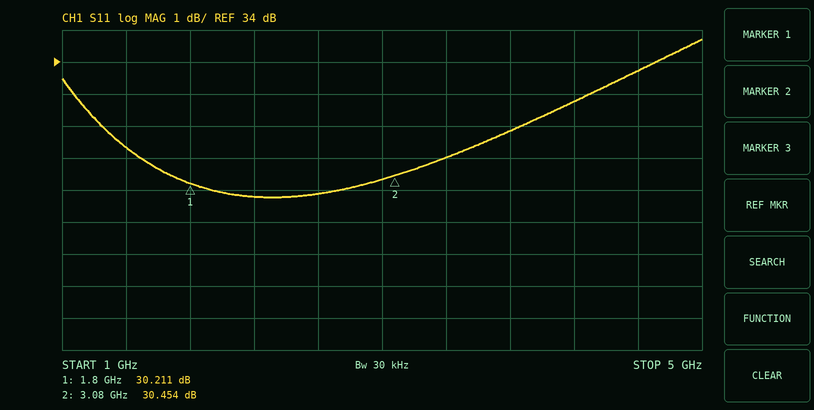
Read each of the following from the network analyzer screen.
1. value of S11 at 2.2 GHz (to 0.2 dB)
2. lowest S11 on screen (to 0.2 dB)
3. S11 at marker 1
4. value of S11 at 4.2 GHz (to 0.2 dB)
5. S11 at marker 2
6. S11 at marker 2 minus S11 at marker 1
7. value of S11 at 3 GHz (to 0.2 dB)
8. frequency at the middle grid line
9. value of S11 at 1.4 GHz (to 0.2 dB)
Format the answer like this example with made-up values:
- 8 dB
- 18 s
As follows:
- 29.8 dB
- 29.8 dB
- 30.211 dB
- 32.8 dB
- 30.454 dB
- 0.243 dB
- 30.4 dB
- 3 GHz
- 31.4 dB
